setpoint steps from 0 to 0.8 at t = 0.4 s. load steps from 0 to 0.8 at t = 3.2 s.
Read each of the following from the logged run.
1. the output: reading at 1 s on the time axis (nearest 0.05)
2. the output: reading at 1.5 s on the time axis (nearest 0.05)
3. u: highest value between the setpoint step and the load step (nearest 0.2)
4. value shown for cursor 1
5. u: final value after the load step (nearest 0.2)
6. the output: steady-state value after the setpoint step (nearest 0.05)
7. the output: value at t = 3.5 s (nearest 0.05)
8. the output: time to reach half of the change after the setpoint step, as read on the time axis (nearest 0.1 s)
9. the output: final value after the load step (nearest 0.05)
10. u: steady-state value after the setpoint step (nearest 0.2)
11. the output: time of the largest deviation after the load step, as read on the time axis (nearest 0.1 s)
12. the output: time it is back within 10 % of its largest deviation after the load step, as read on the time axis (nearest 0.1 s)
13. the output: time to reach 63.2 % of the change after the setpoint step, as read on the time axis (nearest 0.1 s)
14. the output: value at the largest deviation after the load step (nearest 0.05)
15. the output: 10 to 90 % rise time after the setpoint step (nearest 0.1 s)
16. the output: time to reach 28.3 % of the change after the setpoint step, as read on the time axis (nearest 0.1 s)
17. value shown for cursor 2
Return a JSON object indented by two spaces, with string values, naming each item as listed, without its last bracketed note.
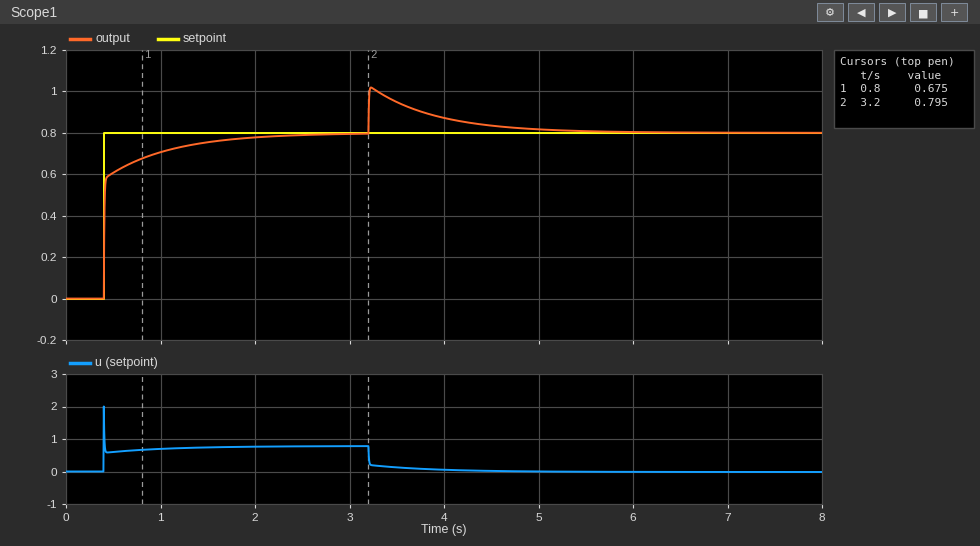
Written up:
{
  "the output: reading at 1 s on the time axis": "0.70",
  "the output: reading at 1.5 s on the time axis": "0.75",
  "u: highest value between the setpoint step and the load step": "2.0",
  "value shown for cursor 1": "0.675",
  "u: final value after the load step": "0.0",
  "the output: steady-state value after the setpoint step": "0.80",
  "the output: value at t = 3.5 s": "0.95",
  "the output: time to reach half of the change after the setpoint step, as read on the time axis": "0.4 s",
  "the output: final value after the load step": "0.80",
  "u: steady-state value after the setpoint step": "0.8",
  "the output: time of the largest deviation after the load step, as read on the time axis": "3.2 s",
  "the output: time it is back within 10 % of its largest deviation after the load step, as read on the time axis": "4.8 s",
  "the output: time to reach 63.2 % of the change after the setpoint step, as read on the time axis": "0.4 s",
  "the output: value at the largest deviation after the load step": "1.00",
  "the output: 10 to 90 % rise time after the setpoint step": "0.7 s",
  "the output: time to reach 28.3 % of the change after the setpoint step, as read on the time axis": "0.4 s",
  "value shown for cursor 2": "0.795"
}
